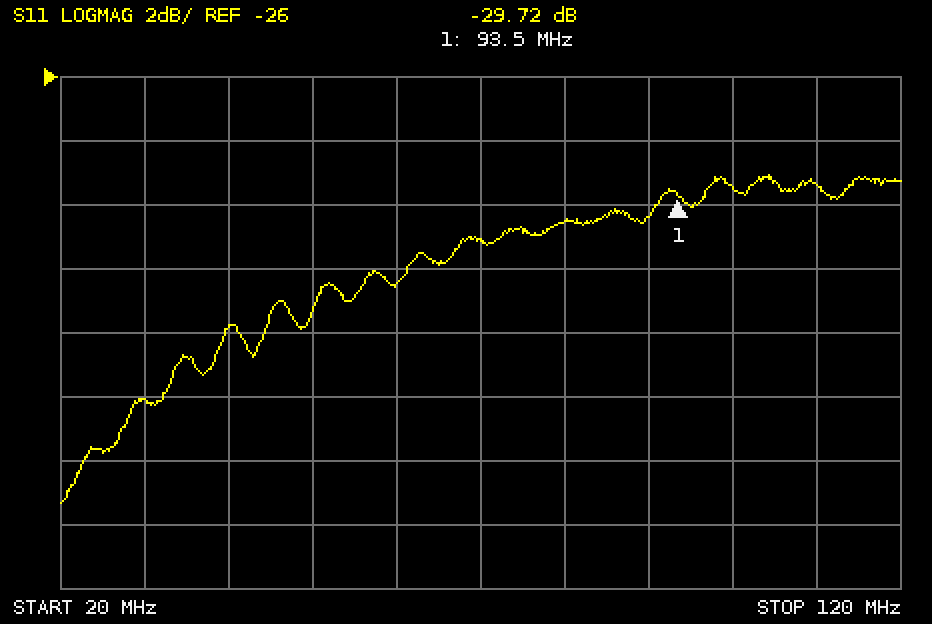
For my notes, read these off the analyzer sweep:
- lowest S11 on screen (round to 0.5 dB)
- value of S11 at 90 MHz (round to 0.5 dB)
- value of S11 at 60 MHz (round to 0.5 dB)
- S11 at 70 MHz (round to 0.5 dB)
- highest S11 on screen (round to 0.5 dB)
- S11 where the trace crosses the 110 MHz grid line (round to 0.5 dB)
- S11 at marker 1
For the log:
-39.5 dB
-30.5 dB
-32.5 dB
-31.0 dB
-29.0 dB
-29.5 dB
-29.72 dB
